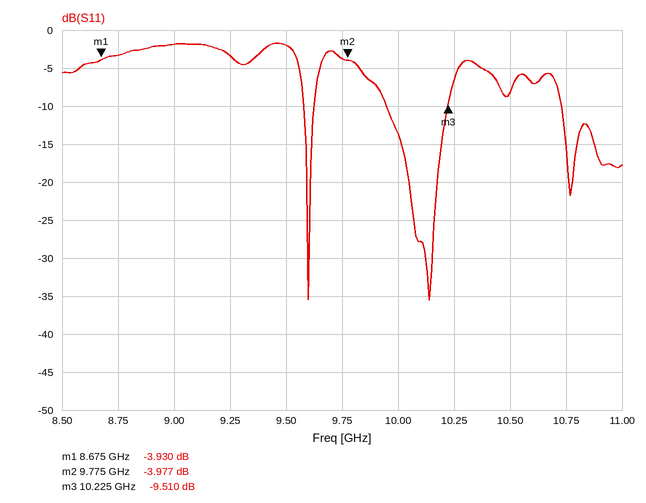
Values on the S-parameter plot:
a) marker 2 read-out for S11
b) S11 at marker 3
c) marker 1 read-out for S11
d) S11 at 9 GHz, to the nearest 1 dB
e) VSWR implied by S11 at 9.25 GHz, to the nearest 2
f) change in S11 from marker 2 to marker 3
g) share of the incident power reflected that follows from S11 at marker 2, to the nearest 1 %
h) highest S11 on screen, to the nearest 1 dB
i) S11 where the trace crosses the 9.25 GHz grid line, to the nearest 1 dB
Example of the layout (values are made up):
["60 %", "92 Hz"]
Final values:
["-3.977 dB", "-9.510 dB", "-3.930 dB", "-2 dB", "6", "-5.533 dB", "40 %", "-2 dB", "-3 dB"]
